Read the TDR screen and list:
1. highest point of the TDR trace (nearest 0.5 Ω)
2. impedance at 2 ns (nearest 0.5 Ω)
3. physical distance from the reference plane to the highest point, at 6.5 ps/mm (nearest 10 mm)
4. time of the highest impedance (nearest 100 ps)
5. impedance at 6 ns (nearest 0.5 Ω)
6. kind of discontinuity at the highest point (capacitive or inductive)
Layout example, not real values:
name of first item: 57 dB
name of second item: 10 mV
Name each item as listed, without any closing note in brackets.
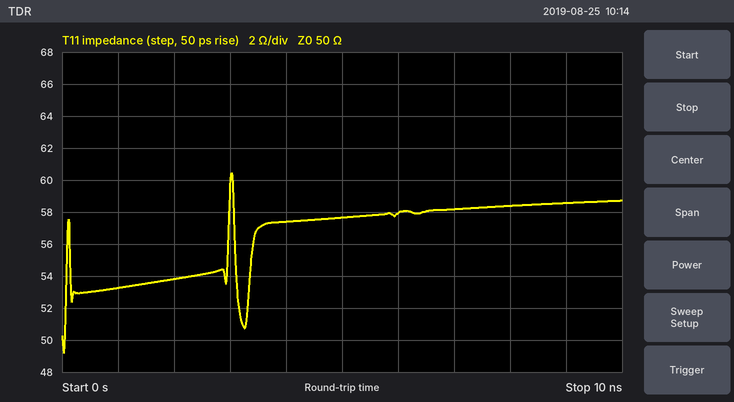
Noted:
highest point of the TDR trace: 60.5 Ω
impedance at 2 ns: 54.0 Ω
physical distance from the reference plane to the highest point, at 6.5 ps/mm: 230 mm
time of the highest impedance: 3.0 ns
impedance at 6 ns: 58.0 Ω
kind of discontinuity at the highest point: inductive
